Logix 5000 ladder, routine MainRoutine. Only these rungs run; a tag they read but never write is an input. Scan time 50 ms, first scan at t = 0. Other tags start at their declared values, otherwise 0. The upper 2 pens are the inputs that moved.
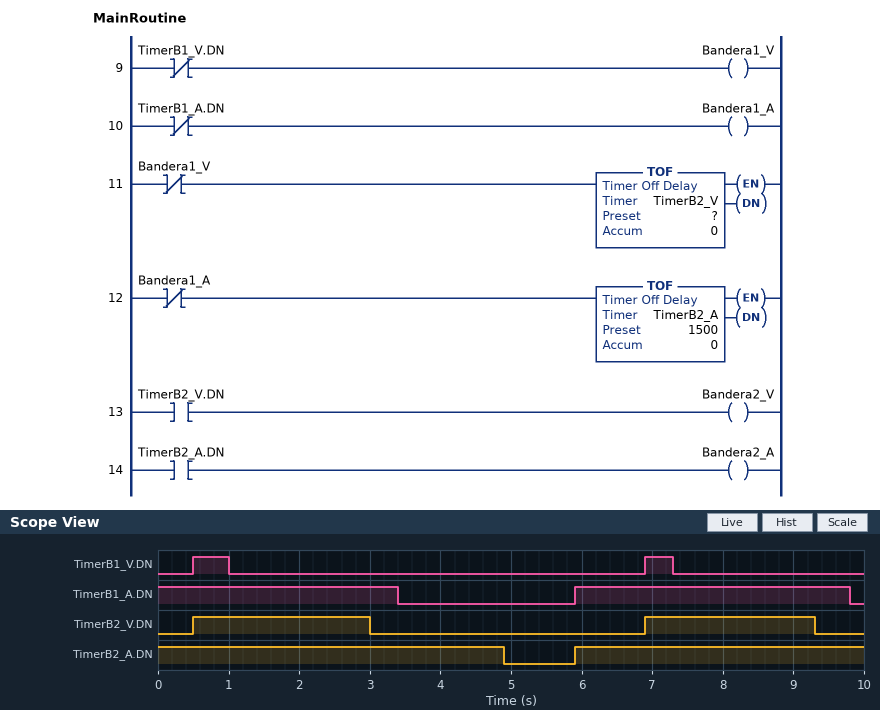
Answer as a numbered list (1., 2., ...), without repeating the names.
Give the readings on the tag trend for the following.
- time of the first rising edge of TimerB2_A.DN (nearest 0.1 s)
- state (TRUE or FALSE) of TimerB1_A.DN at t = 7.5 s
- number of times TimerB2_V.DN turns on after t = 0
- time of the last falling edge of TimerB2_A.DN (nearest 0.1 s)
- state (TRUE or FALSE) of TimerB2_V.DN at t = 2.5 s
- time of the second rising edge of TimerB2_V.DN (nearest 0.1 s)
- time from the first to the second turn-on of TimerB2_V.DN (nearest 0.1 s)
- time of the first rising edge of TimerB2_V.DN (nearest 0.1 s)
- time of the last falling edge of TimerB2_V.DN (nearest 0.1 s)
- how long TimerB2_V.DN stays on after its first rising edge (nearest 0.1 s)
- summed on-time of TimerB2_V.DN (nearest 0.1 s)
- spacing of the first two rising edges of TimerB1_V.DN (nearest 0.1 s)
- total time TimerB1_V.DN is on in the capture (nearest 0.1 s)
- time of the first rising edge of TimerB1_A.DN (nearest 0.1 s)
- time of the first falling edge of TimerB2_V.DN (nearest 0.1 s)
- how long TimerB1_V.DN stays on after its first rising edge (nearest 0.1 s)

1. 5.9 s
2. TRUE
3. 2
4. 4.9 s
5. TRUE
6. 6.9 s
7. 6.4 s
8. 0.5 s
9. 9.3 s
10. 2.5 s
11. 4.9 s
12. 6.4 s
13. 0.9 s
14. 5.9 s
15. 3.0 s
16. 0.5 s
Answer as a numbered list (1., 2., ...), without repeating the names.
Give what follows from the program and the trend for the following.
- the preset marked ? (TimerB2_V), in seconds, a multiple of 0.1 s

1. 2.0 s
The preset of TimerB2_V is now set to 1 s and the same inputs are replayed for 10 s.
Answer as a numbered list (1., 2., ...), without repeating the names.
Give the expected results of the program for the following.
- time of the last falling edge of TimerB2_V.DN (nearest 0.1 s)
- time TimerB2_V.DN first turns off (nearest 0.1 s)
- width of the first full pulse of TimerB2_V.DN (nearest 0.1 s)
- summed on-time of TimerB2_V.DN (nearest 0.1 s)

1. 8.3 s
2. 2.0 s
3. 1.5 s
4. 2.9 s
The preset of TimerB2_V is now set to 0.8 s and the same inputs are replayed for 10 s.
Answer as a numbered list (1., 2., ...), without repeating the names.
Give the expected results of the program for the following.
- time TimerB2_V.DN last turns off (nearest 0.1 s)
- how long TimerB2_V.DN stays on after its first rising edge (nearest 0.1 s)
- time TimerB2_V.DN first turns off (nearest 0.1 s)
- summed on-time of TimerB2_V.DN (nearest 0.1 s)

1. 8.1 s
2. 1.3 s
3. 1.8 s
4. 2.5 s
